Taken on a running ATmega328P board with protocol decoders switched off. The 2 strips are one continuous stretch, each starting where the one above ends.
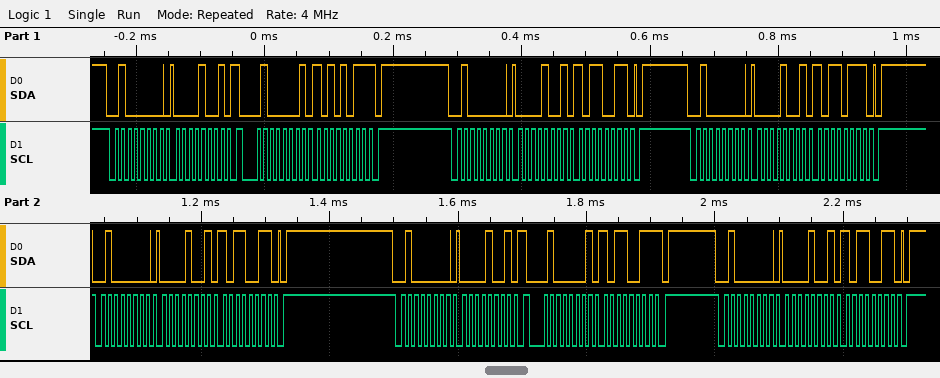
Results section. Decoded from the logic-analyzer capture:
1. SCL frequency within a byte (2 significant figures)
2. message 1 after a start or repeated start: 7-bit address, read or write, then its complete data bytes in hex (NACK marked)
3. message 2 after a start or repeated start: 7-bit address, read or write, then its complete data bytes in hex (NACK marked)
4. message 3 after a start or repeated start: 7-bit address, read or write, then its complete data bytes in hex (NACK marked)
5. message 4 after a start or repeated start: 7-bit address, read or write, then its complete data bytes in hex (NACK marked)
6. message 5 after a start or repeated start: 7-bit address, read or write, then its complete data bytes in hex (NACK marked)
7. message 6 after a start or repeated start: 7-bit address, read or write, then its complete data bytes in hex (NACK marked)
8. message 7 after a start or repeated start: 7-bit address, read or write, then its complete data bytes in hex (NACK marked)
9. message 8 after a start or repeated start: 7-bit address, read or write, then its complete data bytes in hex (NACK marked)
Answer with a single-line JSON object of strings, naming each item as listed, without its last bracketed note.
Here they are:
{"SCL frequency within a byte": "100 kHz", "message 1 after a start or repeated start: 7-bit address, read or write, then its complete data bytes in hex": "0x20 write: 09", "message 2 after a start or repeated start: 7-bit address, read or write, then its complete data bytes in hex": "0x20 read: AB NACK", "message 3 after a start or repeated start: 7-bit address, read or write, then its complete data bytes in hex": "0x20 write: 09 B3", "message 4 after a start or repeated start: 7-bit address, read or write, then its complete data bytes in hex": "0x20 write: 09 B7", "message 5 after a start or repeated start: 7-bit address, read or write, then its complete data bytes in hex": "0x20 write: 09 B3", "message 6 after a start or repeated start: 7-bit address, read or write, then its complete data bytes in hex": "0x20 write: 09", "message 7 after a start or repeated start: 7-bit address, read or write, then its complete data bytes in hex": "0x20 read: B3 NACK", "message 8 after a start or repeated start: 7-bit address, read or write, then its complete data bytes in hex": "0x20 write: 09 B3"}
